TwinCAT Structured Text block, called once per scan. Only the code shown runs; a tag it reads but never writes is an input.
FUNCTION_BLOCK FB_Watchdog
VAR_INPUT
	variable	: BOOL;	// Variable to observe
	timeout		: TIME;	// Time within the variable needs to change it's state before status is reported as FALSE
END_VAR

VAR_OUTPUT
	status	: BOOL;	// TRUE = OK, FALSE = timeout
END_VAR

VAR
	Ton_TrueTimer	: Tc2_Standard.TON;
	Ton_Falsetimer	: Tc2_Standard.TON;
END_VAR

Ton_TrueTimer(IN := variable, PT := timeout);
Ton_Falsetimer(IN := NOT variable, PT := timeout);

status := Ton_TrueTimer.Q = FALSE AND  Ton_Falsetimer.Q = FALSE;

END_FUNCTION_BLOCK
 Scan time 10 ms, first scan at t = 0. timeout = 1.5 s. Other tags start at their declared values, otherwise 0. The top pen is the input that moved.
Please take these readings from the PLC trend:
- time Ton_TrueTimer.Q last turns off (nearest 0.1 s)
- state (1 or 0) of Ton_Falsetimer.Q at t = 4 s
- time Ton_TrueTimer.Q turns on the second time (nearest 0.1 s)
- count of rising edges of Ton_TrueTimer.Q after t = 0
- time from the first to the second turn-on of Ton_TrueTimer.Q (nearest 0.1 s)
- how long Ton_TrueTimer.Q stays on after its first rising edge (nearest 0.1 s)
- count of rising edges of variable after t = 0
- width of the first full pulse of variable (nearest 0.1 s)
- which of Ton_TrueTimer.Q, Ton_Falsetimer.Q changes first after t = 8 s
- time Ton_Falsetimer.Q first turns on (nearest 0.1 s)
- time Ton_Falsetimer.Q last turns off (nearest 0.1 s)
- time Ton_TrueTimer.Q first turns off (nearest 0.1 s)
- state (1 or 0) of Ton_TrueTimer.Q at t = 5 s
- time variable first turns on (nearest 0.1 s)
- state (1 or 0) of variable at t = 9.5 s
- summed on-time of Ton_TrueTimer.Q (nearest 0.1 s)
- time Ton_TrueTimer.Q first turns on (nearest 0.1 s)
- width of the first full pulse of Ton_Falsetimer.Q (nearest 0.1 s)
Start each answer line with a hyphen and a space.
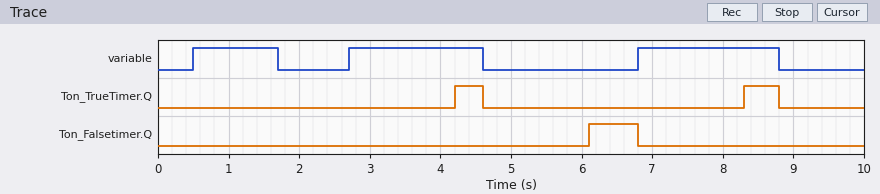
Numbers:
- 8.8 s
- 0
- 8.3 s
- 2
- 4.1 s
- 0.4 s
- 3
- 1.2 s
- Ton_TrueTimer.Q
- 6.1 s
- 6.8 s
- 4.6 s
- 0
- 0.5 s
- 0
- 0.9 s
- 4.2 s
- 0.7 s
